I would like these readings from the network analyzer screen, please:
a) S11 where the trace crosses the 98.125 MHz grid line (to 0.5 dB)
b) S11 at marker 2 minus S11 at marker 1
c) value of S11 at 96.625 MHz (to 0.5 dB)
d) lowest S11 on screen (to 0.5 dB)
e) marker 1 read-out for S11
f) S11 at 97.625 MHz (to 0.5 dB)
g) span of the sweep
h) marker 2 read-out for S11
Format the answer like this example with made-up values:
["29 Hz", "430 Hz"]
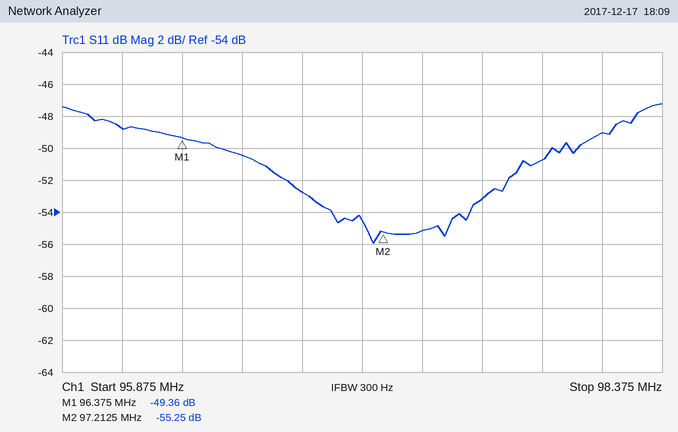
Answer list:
["-49.0 dB", "-5.89 dB", "-50.5 dB", "-56.0 dB", "-49.36 dB", "-53.0 dB", "2.5 MHz", "-55.25 dB"]
